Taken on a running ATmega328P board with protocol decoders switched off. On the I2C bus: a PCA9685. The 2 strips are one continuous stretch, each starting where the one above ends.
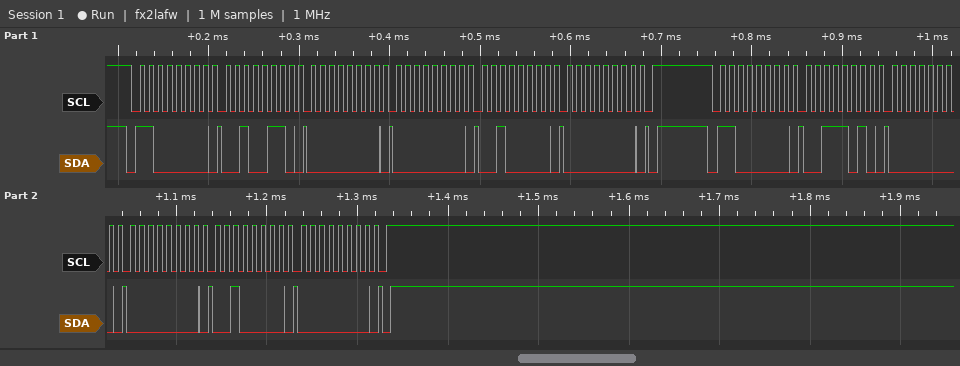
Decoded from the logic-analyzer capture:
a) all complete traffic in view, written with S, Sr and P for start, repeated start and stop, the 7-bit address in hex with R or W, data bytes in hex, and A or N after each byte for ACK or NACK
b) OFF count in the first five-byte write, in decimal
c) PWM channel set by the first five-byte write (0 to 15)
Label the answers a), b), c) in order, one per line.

a) S 60W A 26 A 00 A 00 A 20 A 00 A P S 60W A 3A A 00 A 00 A 20 A 00 A P
b) 32
c) 8
